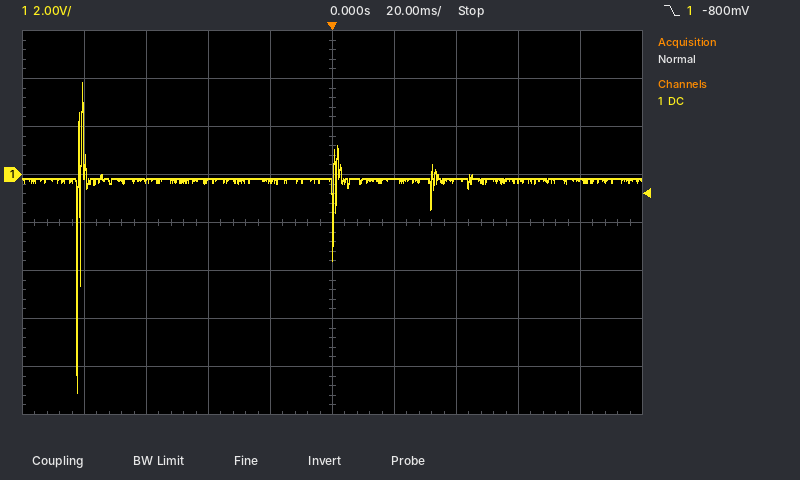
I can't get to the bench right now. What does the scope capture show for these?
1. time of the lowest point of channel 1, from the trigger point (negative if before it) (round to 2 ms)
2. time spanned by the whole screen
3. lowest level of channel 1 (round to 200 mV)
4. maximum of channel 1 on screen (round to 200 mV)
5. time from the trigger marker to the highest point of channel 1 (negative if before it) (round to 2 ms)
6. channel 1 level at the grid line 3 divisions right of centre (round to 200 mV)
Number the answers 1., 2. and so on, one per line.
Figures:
1. -82 ms
2. 200 ms
3. -9.0 V
4. 3.8 V
5. -80 ms
6. -200 mV
